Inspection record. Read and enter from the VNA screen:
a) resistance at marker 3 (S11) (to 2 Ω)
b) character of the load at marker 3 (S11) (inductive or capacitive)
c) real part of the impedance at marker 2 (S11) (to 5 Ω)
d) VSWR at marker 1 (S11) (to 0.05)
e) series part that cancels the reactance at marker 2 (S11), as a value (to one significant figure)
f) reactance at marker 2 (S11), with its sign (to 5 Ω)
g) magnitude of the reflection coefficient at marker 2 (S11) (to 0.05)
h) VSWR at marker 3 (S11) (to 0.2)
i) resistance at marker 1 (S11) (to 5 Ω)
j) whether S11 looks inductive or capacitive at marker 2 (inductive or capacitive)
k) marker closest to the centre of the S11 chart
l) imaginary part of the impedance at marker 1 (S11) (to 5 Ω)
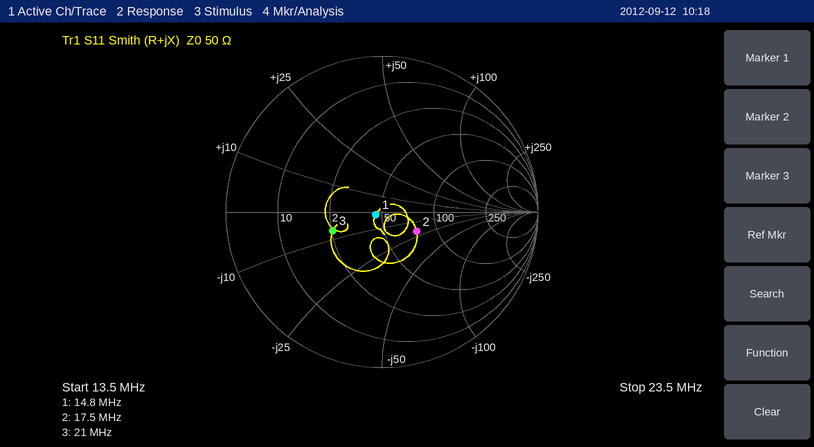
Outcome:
26 Ω
capacitive
75 Ω
1.10
200 nH
-20 Ω
0.25
2.0
45 Ω
capacitive
marker 1
0 Ω
